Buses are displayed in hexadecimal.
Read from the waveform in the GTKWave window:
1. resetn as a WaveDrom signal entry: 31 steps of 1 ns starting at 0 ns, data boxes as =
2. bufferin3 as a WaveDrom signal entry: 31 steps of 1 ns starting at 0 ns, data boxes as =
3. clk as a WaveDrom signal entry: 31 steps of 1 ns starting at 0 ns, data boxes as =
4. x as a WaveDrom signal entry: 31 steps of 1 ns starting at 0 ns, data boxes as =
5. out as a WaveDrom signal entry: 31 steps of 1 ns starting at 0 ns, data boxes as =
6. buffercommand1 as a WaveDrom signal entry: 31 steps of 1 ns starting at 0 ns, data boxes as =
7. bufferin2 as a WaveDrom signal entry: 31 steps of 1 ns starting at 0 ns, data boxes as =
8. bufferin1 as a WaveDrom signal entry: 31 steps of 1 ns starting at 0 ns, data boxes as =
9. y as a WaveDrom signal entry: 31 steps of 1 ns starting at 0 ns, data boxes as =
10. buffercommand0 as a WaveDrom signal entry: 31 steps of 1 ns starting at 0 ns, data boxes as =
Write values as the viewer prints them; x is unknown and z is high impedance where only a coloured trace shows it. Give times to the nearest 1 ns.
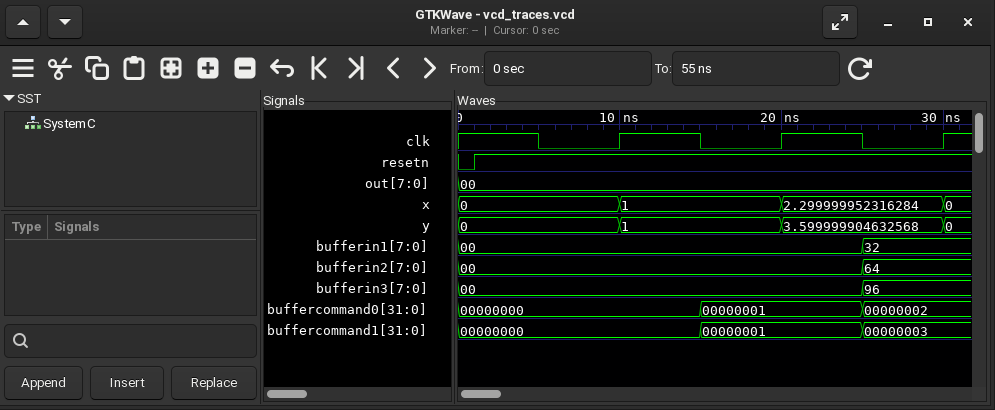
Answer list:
{name: 'resetn', wave: '01.............................'}
{name: 'bufferin3', wave: '=........................=.....', data: '00 96'}
{name: 'clk', wave: '1....0....1....0....1....0....1'}
{name: 'x', wave: '=.........=.........=.........=', data: '0 1 2.299999952316284 0'}
{name: 'out', wave: '=..............................', data: '00'}
{name: 'buffercommand1', wave: '=..............=.........=.....', data: '00000000 00000001 00000003'}
{name: 'bufferin2', wave: '=........................=.....', data: '00 64'}
{name: 'bufferin1', wave: '=........................=.....', data: '00 32'}
{name: 'y', wave: '=.........=.........=.........=', data: '0 1 3.599999904632568 0'}
{name: 'buffercommand0', wave: '=..............=.........=.....', data: '00000000 00000001 00000002'}
